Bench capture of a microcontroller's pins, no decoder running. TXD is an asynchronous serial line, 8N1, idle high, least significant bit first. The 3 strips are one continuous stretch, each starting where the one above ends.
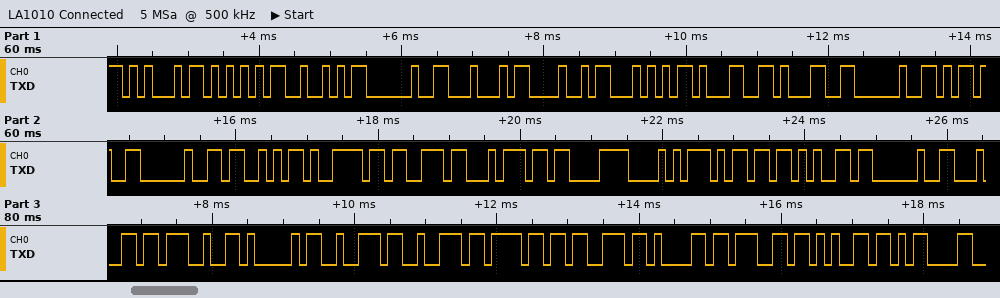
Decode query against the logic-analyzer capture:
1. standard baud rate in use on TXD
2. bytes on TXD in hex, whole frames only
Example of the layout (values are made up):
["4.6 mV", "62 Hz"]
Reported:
["9600 baud", "45 55 52 20 44 48 54 31 31 20 2D 20 53 79 73 74 C3 A8 6D 65 20 64 27 41 72 72 6F 73 61 67 65 0D"]
